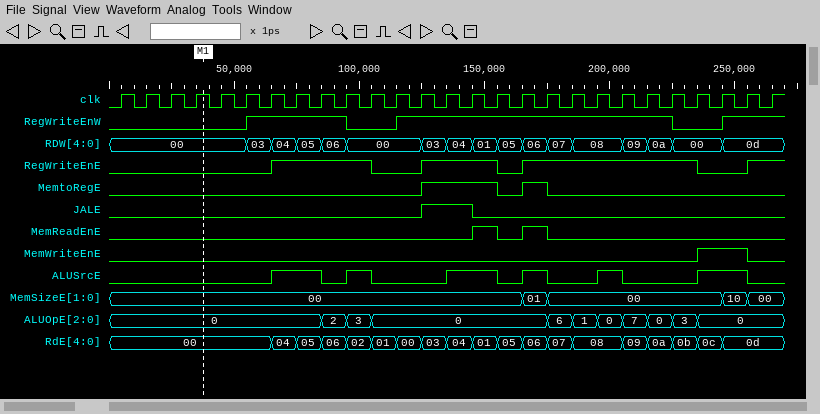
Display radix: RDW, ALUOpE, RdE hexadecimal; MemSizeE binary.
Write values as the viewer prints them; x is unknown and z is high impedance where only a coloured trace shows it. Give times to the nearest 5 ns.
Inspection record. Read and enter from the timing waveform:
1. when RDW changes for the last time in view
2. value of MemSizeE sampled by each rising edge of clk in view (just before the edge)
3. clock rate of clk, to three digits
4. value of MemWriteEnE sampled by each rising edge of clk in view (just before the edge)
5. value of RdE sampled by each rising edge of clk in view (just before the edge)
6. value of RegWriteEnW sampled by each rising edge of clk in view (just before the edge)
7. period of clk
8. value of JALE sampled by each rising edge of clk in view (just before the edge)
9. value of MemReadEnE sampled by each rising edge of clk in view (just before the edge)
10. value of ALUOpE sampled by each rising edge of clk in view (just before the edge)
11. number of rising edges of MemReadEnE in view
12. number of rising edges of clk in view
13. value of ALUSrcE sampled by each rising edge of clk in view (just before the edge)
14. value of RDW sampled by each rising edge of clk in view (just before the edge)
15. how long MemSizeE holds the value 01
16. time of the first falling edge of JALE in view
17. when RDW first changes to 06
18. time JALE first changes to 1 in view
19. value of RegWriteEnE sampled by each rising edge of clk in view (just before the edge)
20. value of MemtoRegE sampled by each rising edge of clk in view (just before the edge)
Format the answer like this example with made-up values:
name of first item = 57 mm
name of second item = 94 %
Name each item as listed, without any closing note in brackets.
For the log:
when RDW changes for the last time in view = 245 ns
value of MemSizeE sampled by each rising edge of clk in view = 00, 00, 00, 00, 00, 00, 00, 00, 00, 00, 00, 00, 00, 00, 00, 00, 00, 01, 00, 00, 00, 00, 00, 00, 00, 10, 00
clock rate of clk, to three digits = 100 MHz
value of MemWriteEnE sampled by each rising edge of clk in view = 0 0 0 0 0 0 0 0 0 0 0 0 0 0 0 0 0 0 0 0 0 0 0 0 1 1 0
value of RdE sampled by each rising edge of clk in view = 00, 00, 00, 00, 00, 00, 00, 04, 05, 06, 02, 01, 00, 03, 04, 01, 05, 06, 07, 08, 08, 09, 0a, 0b, 0c, 0d, 0d
value of RegWriteEnW sampled by each rising edge of clk in view = 0 0 0 0 0 0 1 1 1 1 0 0 1 1 1 1 1 1 1 1 1 1 1 0 0 1 1
period of clk = 10 ns
value of JALE sampled by each rising edge of clk in view = 0 0 0 0 0 0 0 0 0 0 0 0 0 1 1 0 0 0 0 0 0 0 0 0 0 0 0
value of MemReadEnE sampled by each rising edge of clk in view = 0 0 0 0 0 0 0 0 0 0 0 0 0 0 0 1 0 1 0 0 0 0 0 0 0 0 0
value of ALUOpE sampled by each rising edge of clk in view = 0, 0, 0, 0, 0, 0, 0, 0, 0, 2, 3, 0, 0, 0, 0, 0, 0, 0, 6, 1, 0, 7, 0, 3, 0, 0, 0
number of rising edges of MemReadEnE in view = 2
number of rising edges of clk in view = 27
value of ALUSrcE sampled by each rising edge of clk in view = 0 0 0 0 0 0 0 1 1 0 1 0 0 0 1 1 0 1 0 0 1 0 0 0 1 1 0
value of RDW sampled by each rising edge of clk in view = 00, 00, 00, 00, 00, 00, 03, 04, 05, 06, 00, 00, 00, 03, 04, 01, 05, 06, 07, 08, 08, 09, 0a, 00, 00, 0d, 0d
how long MemSizeE holds the value 01 = 10 ns
time of the first falling edge of JALE in view = 145 ns
when RDW first changes to 06 = 85 ns
time JALE first changes to 1 in view = 125 ns
value of RegWriteEnE sampled by each rising edge of clk in view = 0 0 0 0 0 0 0 1 1 1 1 0 0 1 1 1 0 1 1 1 1 1 1 1 0 0 1
value of MemtoRegE sampled by each rising edge of clk in view = 0 0 0 0 0 0 0 0 0 0 0 0 0 1 1 1 0 1 0 0 0 0 0 0 0 0 0
